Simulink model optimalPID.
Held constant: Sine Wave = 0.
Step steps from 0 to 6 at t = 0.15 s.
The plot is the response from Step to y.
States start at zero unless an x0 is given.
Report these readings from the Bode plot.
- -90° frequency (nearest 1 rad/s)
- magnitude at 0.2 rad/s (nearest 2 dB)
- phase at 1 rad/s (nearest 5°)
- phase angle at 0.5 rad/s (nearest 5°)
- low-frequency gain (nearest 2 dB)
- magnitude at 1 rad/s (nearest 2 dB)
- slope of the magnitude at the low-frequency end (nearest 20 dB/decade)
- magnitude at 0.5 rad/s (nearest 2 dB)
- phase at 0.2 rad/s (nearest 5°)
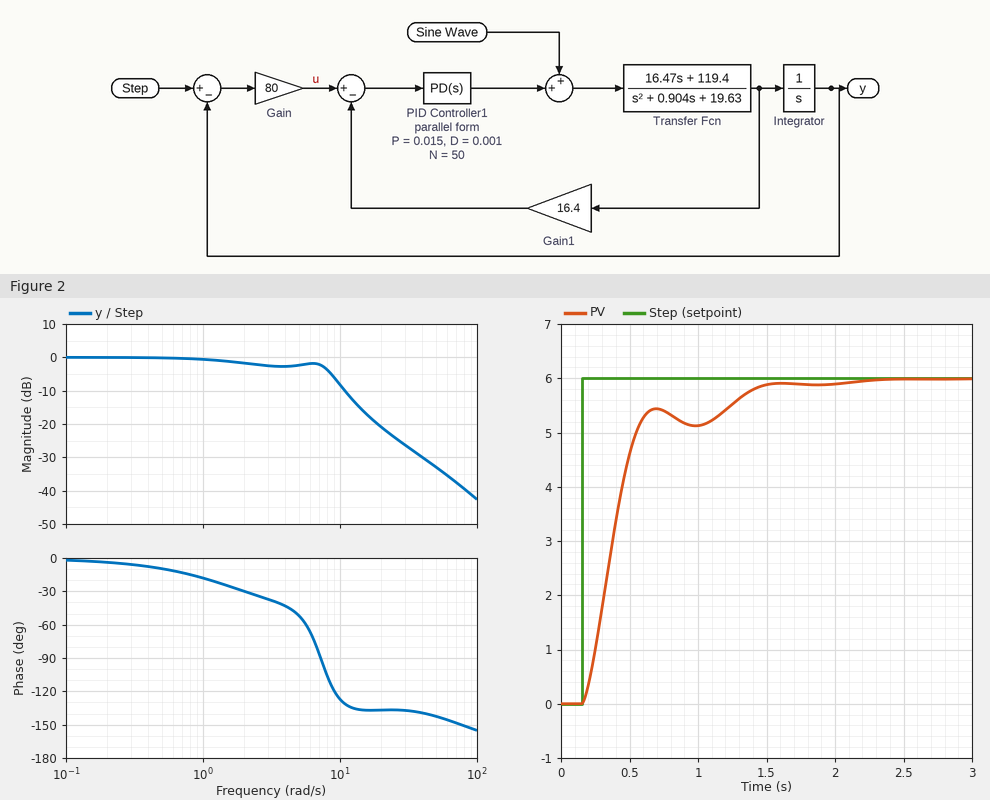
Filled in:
7 rad/s
0 dB
-20°
-10°
0 dB
0 dB
0 dB/decade
0 dB
-5°
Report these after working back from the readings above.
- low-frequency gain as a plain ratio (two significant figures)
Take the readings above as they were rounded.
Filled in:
1.0
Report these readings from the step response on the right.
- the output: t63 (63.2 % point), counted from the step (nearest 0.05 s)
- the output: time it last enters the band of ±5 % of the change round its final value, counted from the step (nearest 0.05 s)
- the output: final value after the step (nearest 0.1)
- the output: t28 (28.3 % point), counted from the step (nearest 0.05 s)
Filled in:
0.30 s
1.20 s
6.0
0.15 s
